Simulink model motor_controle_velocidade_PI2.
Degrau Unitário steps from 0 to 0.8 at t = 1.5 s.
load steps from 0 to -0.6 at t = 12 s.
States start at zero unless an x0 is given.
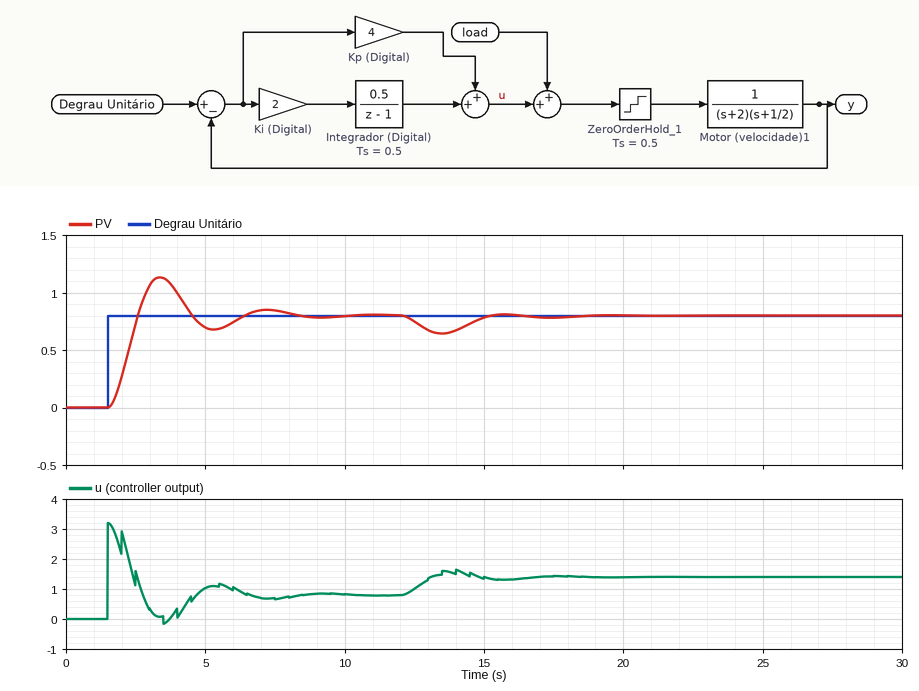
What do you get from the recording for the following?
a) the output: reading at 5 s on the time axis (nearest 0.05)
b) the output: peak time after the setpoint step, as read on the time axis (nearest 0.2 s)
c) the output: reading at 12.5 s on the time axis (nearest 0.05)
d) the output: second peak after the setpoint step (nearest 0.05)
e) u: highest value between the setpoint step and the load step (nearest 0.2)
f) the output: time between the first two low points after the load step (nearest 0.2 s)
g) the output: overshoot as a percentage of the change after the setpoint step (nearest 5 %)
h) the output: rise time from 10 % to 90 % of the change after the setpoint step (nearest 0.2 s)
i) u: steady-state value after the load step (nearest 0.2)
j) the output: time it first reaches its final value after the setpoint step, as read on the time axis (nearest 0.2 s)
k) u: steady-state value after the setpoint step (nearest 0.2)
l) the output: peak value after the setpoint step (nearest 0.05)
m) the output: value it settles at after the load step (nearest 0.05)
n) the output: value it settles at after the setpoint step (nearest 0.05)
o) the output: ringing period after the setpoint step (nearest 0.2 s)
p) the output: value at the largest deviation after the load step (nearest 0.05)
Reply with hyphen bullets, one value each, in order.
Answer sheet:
- 0.70
- 3.4 s
- 0.75
- 0.85
- 3.2
- 3.8 s
- 40 %
- 0.8 s
- 1.4
- 2.6 s
- 0.8
- 1.15
- 0.80
- 0.80
- 3.8 s
- 0.65
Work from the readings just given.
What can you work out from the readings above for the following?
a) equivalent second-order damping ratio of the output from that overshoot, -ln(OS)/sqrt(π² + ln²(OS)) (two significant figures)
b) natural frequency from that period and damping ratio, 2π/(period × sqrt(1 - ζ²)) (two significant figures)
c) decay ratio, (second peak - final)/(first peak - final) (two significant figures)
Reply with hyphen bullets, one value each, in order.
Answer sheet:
- 0.28
- 1.7 rad/s
- 0.14
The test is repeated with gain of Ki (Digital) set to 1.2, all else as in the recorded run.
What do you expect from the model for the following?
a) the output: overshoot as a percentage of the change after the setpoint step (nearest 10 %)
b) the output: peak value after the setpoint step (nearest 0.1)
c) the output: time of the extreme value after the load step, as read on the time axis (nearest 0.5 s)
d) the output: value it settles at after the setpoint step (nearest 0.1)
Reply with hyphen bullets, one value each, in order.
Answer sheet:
- 30 %
- 1.0
- 13.5 s
- 0.8
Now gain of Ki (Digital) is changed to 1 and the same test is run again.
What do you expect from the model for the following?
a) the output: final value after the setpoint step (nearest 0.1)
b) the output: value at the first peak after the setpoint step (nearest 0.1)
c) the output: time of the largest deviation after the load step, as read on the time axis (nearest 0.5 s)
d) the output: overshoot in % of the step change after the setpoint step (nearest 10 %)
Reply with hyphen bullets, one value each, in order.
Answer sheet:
- 0.8
- 1.0
- 13.5 s
- 20 %
